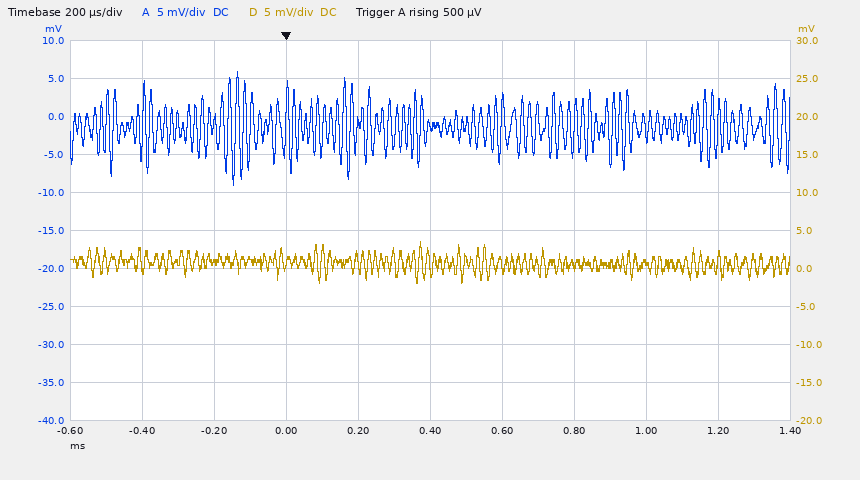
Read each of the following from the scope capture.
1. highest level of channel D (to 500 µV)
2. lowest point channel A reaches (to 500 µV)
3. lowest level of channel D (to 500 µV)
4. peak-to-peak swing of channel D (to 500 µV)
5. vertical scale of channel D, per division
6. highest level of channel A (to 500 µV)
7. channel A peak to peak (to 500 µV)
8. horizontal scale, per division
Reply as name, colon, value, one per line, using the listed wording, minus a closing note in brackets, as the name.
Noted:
highest level of channel D: 3.5 mV
lowest point channel A reaches: -9.0 mV
lowest level of channel D: -2.0 mV
peak-to-peak swing of channel D: 5.5 mV
vertical scale of channel D, per division: 5 mV
highest level of channel A: 6.0 mV
channel A peak to peak: 15.0 mV
horizontal scale, per division: 200 µs
